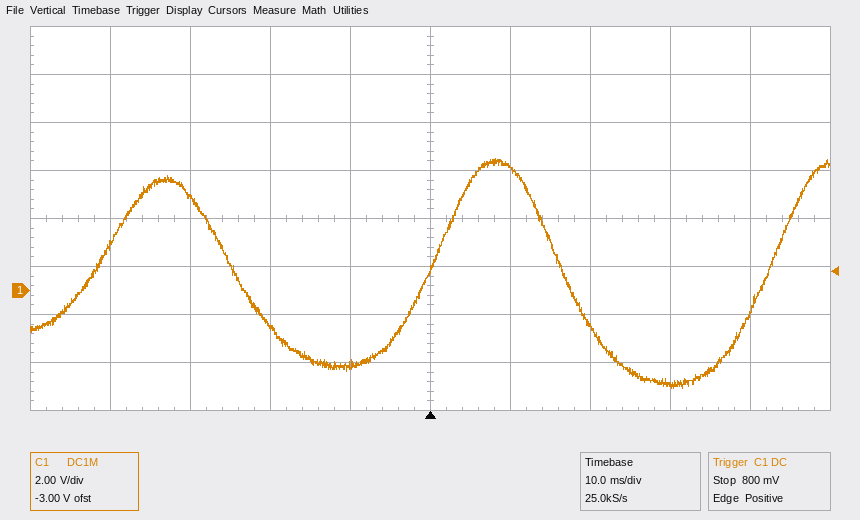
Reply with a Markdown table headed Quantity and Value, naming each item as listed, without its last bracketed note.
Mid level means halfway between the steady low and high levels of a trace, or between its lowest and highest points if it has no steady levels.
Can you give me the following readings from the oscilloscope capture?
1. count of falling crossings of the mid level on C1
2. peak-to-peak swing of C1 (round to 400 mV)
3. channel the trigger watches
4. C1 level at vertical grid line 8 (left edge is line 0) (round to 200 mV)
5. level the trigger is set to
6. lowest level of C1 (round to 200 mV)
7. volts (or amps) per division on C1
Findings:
| Quantity | Value |
|---|---|
| count of falling crossings of the mid level on C1 | 2 |
| peak-to-peak swing of C1 | 9.6 V |
| channel the trigger watches | C1 |
| C1 level at vertical grid line 8 (left edge is line 0) | -4.0 V |
| level the trigger is set to | 800 mV |
| lowest level of C1 | -4.0 V |
| volts (or amps) per division on C1 | 2 V |
